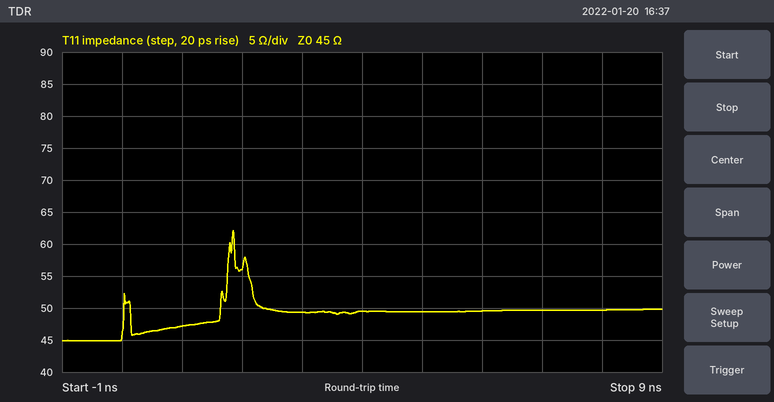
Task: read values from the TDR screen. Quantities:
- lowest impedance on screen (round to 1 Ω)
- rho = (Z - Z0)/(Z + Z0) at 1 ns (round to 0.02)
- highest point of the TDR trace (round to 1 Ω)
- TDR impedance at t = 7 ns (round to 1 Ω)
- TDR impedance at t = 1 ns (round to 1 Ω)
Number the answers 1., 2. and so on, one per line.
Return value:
1. 45 Ω
2. +0.02
3. 62 Ω
4. 50 Ω
5. 47 Ω
